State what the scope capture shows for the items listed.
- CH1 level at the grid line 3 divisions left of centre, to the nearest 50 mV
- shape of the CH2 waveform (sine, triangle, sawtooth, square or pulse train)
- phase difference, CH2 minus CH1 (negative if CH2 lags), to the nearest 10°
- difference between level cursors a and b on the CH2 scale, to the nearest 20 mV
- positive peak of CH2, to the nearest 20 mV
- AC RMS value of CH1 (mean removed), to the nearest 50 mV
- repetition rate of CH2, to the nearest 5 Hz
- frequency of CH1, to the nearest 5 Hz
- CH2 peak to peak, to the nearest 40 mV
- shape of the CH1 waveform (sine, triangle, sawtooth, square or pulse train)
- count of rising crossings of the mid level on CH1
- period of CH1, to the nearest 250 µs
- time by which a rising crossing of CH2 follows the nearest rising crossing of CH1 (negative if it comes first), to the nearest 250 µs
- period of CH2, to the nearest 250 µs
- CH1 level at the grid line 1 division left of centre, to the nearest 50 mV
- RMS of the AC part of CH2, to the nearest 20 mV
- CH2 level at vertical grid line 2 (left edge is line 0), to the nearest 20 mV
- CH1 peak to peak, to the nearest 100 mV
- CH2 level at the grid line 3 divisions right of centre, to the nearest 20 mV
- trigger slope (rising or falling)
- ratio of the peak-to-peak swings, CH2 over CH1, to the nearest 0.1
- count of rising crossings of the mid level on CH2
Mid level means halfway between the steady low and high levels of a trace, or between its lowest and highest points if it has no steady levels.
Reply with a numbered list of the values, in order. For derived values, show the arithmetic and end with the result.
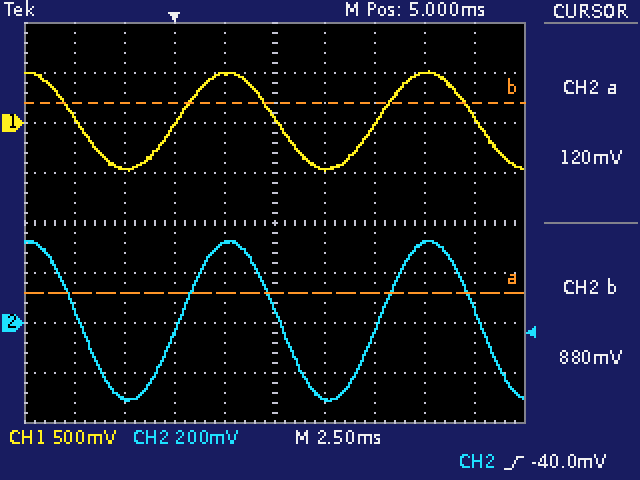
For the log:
1. -450 mV
2. sine
3. −360° × (0.00 ms) / 10.00 ms ≈ 0°
4. 760 mV
5. 320 mV
6. 1.00 V / (2√2) ≈ 354 mV, so 350 mV to the nearest 50 mV
7. 1 / 10.00 ms ≈ 100 Hz
8. 1 / 10.00 ms ≈ 100 Hz
9. 640 mV
10. sine
11. 2
12. 10.00 ms
13. 0.00 ms
14. 10.00 ms
15. 500 mV
16. 640 mV / (2√2) ≈ 226 mV, so 220 mV to the nearest 20 mV
17. -300 mV
18. 1.00 V
19. 320 mV
20. rising
21. 640 mV / 1.00 V ≈ 0.6
22. 2
